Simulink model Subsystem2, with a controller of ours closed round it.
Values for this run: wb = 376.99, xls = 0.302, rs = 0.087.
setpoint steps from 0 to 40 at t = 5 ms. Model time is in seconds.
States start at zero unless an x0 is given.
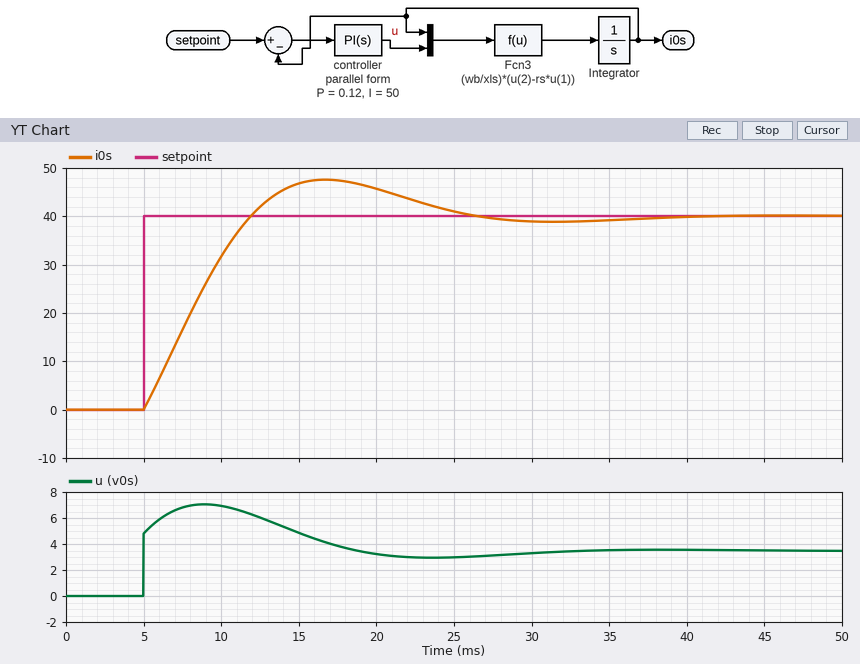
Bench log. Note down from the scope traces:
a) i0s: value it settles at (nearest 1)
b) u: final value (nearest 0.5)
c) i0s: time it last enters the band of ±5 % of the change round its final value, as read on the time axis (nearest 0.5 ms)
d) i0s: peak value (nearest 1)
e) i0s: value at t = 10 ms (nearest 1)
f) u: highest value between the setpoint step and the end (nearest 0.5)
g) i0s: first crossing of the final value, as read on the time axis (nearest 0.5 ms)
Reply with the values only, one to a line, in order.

40
3.5
24.0 ms
48
32
7.0
12.0 ms
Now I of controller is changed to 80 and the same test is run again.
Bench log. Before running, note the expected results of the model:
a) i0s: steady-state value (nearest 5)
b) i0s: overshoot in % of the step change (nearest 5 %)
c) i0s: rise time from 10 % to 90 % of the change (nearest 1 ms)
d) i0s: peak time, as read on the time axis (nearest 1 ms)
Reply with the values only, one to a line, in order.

40
30 %
4 ms
14 ms
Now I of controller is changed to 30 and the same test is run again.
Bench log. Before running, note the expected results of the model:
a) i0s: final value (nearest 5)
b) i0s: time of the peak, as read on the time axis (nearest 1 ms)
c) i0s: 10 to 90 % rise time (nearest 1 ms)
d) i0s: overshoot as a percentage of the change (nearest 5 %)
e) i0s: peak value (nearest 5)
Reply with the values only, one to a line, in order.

40
21 ms
7 ms
10 %
45
